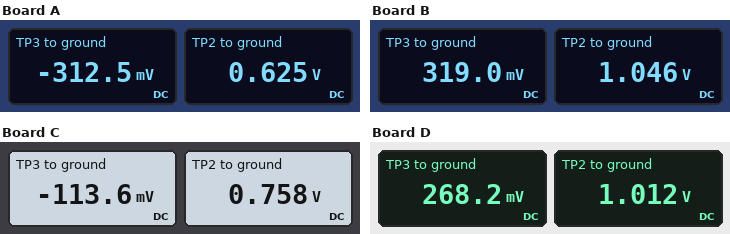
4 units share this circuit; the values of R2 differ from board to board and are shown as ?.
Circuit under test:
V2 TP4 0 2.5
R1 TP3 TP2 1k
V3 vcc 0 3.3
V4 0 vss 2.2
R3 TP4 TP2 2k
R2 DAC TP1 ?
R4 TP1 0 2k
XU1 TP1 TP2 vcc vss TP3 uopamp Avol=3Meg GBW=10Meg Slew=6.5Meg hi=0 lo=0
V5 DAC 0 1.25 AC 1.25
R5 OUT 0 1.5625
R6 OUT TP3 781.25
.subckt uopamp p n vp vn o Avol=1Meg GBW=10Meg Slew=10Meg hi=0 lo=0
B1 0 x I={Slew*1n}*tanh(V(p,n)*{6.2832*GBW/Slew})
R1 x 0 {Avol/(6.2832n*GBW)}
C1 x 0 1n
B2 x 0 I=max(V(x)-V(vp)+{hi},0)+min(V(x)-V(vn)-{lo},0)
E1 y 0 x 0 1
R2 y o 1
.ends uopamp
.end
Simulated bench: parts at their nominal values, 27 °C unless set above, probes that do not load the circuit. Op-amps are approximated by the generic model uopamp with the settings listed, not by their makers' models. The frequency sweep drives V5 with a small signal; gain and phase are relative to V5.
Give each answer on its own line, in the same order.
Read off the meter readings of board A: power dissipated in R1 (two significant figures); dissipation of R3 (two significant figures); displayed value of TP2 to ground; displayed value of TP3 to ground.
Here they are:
880 µW
1.8 mW
0.625 V
-312.5 mV
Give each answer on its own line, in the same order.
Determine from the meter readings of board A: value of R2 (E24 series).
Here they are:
2 kΩ
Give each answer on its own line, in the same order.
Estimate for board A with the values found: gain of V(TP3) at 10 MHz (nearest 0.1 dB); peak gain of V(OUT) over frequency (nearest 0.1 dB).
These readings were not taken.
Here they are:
-7.6 dB
-56.5 dB
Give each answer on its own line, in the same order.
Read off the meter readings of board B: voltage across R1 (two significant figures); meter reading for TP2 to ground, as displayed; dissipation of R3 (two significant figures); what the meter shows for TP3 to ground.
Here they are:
730 mV
1.046 V
1.1 mW
319.0 mV
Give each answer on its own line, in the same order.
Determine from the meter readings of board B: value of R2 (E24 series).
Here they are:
390 Ω
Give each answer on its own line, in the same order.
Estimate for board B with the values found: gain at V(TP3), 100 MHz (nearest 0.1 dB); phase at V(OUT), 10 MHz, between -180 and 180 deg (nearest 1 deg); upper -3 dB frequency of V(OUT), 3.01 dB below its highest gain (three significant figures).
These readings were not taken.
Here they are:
-21.6 dB
-56 deg
6.66 MHz
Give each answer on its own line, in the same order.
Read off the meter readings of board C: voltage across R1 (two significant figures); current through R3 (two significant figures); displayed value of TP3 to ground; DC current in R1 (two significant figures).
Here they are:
870 mV
870 µA
-113.6 mV
870 µA
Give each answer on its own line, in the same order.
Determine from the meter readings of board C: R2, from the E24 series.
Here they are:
1.3 kΩ
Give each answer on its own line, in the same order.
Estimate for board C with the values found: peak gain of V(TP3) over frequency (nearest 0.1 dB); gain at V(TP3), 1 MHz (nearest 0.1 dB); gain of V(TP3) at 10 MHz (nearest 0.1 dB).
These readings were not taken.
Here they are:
-0.8 dB
-0.9 dB
-6.0 dB
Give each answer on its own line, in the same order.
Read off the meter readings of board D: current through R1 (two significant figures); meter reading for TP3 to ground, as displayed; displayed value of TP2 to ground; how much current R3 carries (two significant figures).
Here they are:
740 µA
268.2 mV
1.012 V
740 µA
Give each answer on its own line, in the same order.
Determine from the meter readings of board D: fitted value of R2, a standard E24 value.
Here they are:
470 Ω
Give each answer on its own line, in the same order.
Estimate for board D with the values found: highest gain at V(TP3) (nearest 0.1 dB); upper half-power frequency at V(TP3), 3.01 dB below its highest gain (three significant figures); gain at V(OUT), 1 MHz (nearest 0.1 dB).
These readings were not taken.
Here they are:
1.7 dB
6.66 MHz
-52.4 dB
